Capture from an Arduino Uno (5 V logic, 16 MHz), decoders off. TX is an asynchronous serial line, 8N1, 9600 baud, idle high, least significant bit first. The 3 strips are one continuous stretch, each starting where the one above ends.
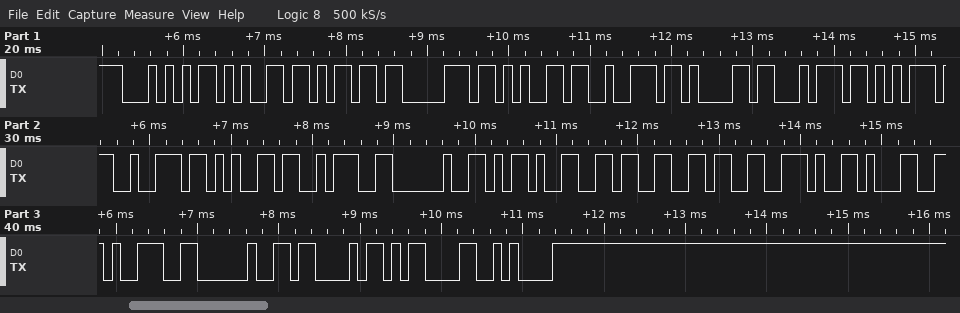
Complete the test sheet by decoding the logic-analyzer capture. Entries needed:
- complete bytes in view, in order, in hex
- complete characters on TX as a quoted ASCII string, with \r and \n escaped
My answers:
54 65 6D 70 65 72 61 74 75 72 65 3A 20 2D 36 36 2E 31 39 20 43 0D 0A
"Temperature: -66.19 C\r\n"
